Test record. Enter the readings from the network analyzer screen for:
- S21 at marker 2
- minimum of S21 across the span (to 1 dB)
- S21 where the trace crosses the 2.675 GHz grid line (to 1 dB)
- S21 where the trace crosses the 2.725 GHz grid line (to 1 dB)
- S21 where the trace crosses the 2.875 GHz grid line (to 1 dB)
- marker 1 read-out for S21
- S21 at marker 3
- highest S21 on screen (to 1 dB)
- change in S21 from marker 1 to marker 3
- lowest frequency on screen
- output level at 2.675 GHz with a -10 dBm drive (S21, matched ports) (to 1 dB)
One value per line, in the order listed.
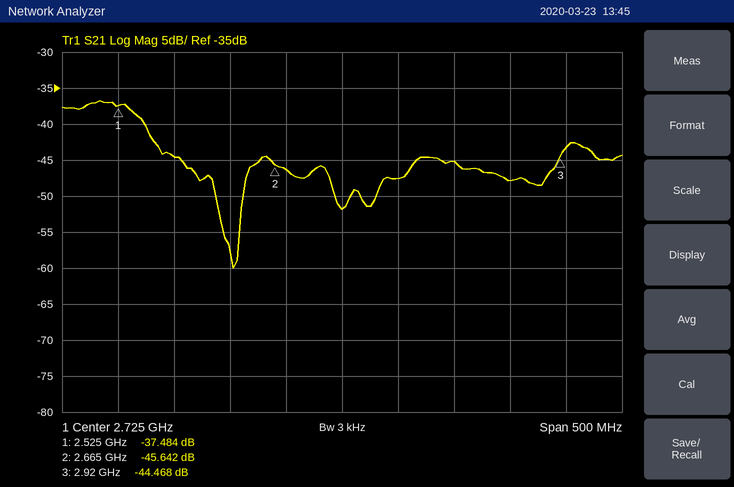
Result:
-45.642 dB
-60 dB
-46 dB
-52 dB
-48 dB
-37.484 dB
-44.468 dB
-37 dB
-6.984 dB
2.475 GHz
-56 dBm
